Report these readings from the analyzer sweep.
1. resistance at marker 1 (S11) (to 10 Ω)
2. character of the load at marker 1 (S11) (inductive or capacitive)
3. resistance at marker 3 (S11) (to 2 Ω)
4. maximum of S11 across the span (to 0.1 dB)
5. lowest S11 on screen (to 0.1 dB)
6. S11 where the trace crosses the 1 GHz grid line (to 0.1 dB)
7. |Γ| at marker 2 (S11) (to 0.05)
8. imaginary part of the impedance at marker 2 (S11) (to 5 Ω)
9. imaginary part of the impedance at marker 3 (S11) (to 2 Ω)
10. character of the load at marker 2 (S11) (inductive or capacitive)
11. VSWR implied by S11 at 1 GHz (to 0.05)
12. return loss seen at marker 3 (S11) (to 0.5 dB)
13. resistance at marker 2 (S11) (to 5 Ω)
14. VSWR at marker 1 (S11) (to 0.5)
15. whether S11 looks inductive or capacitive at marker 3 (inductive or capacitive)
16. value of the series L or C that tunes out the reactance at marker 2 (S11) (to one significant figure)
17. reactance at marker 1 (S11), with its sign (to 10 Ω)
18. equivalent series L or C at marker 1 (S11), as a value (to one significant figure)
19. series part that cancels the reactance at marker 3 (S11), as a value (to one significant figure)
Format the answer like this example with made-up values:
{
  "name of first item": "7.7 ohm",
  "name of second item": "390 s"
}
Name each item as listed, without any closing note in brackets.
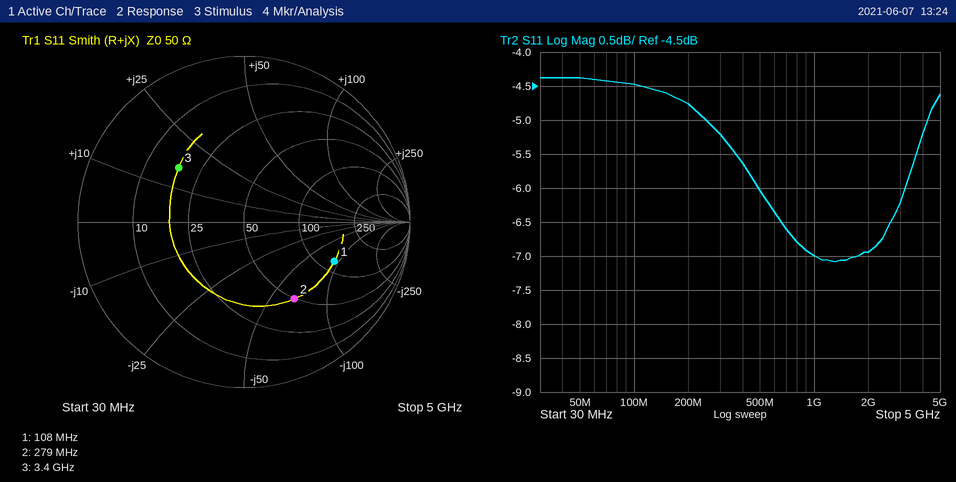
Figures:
{
  "resistance at marker 1 (S11)": "120 Ω",
  "character of the load at marker 1 (S11)": "capacitive",
  "resistance at marker 3 (S11)": "18 Ω",
  "maximum of S11 across the span": "-4.4 dB",
  "lowest S11 on screen": "-7.1 dB",
  "S11 where the trace crosses the 1 GHz grid line": "-7.0 dB",
  "|Γ| at marker 2 (S11)": "0.55",
  "imaginary part of the impedance at marker 2 (S11)": "-65 Ω",
  "imaginary part of the impedance at marker 3 (S11)": "+16 Ω",
  "character of the load at marker 2 (S11)": "capacitive",
  "VSWR implied by S11 at 1 GHz": "2.60",
  "return loss seen at marker 3 (S11)": "6.0 dB",
  "resistance at marker 2 (S11)": "50 Ω",
  "VSWR at marker 1 (S11)": "4.0",
  "whether S11 looks inductive or capacitive at marker 3": "inductive",
  "value of the series L or C that tunes out the reactance at marker 2 (S11)": "40 nH",
  "reactance at marker 1 (S11), with its sign": "-90 Ω",
  "equivalent series L or C at marker 1 (S11), as a value": "20 pF",
  "series part that cancels the reactance at marker 3 (S11), as a value": "3 pF"
}
